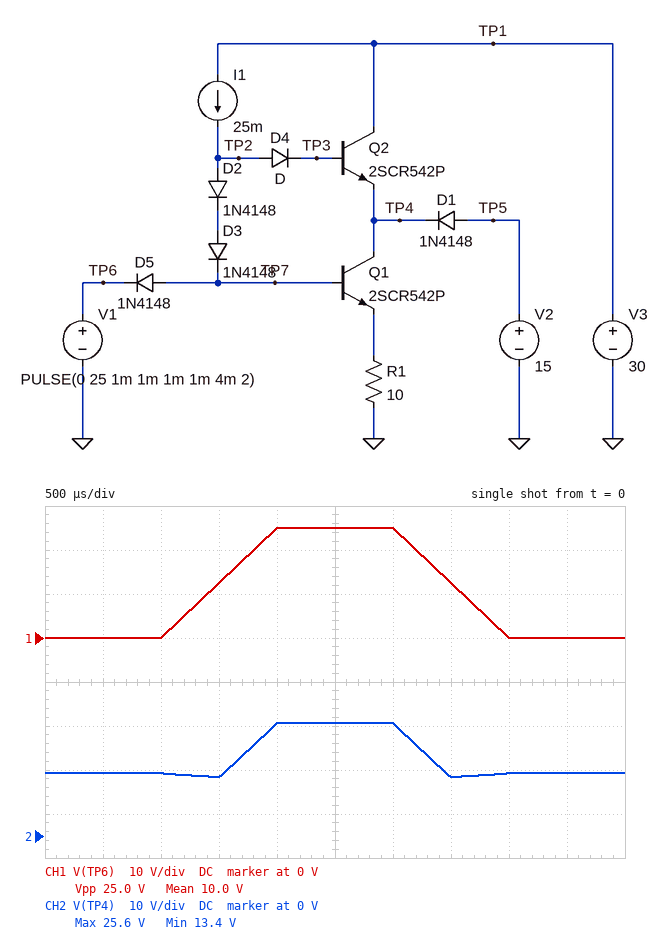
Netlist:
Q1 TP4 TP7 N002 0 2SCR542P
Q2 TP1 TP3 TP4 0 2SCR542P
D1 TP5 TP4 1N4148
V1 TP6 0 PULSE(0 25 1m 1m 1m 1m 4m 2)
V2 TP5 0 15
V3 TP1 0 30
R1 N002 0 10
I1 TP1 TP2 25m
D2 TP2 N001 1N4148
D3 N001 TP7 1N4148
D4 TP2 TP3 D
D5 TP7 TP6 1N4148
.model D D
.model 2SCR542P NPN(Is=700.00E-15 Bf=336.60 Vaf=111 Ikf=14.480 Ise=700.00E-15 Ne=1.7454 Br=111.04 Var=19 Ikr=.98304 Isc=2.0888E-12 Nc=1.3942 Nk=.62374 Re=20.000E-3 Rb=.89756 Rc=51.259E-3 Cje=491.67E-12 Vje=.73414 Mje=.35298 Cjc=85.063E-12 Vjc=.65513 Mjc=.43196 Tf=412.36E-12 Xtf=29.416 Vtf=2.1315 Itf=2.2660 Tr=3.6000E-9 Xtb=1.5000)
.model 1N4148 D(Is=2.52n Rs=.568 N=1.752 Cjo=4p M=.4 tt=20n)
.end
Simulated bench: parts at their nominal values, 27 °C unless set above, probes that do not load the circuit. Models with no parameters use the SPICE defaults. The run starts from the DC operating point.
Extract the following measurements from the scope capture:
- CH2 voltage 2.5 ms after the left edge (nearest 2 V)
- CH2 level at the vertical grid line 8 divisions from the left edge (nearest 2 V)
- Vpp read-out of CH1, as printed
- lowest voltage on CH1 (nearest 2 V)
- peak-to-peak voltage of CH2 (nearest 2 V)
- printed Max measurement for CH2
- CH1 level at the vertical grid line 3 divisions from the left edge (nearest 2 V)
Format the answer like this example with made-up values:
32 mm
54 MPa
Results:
26 V
14 V
25.0 V
0 V
12 V
25.6 V
12 V
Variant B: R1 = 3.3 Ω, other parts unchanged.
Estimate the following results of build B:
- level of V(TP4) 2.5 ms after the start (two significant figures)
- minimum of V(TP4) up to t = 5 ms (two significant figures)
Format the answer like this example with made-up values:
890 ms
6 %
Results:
13 V
12 V
